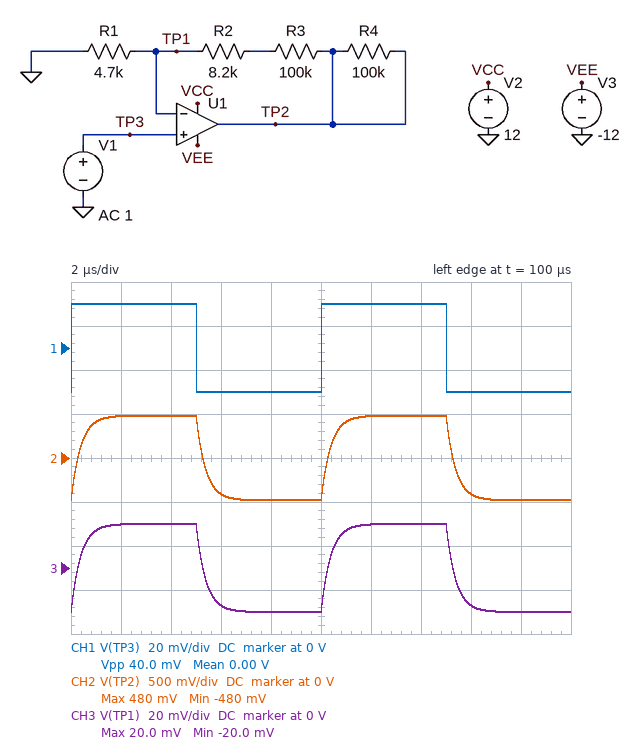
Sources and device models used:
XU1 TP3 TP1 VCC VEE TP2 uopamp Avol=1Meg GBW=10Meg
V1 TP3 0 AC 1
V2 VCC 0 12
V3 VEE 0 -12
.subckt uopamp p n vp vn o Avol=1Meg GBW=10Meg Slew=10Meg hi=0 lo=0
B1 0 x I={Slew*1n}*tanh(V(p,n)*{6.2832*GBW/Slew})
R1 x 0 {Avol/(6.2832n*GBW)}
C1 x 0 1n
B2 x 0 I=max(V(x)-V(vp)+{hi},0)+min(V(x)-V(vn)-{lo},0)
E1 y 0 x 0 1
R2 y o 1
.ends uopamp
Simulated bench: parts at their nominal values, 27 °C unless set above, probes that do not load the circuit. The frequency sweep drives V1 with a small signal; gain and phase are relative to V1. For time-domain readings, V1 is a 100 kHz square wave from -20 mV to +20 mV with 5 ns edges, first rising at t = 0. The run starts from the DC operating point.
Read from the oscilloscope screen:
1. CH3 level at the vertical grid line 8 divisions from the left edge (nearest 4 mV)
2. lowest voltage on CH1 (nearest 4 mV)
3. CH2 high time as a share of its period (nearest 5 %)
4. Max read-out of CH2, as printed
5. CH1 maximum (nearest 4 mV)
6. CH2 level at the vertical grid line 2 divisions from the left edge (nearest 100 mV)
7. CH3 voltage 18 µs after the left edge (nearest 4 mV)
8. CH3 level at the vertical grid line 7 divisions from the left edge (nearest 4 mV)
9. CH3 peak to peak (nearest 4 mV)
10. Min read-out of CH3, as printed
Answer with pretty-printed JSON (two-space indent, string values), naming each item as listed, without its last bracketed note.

{
  "CH3 level at the vertical grid line 8 divisions from the left edge": "-16 mV",
  "lowest voltage on CH1": "-20 mV",
  "CH2 high time as a share of its period": "50 %",
  "Max read-out of CH2, as printed": "480 mV",
  "CH1 maximum": "20 mV",
  "CH2 level at the vertical grid line 2 divisions from the left edge": "500 mV",
  "CH3 voltage 18 µs after the left edge": "-20 mV",
  "CH3 level at the vertical grid line 7 divisions from the left edge": "20 mV",
  "CH3 peak to peak": "40 mV",
  "Min read-out of CH3, as printed": "-20.0 mV"
}
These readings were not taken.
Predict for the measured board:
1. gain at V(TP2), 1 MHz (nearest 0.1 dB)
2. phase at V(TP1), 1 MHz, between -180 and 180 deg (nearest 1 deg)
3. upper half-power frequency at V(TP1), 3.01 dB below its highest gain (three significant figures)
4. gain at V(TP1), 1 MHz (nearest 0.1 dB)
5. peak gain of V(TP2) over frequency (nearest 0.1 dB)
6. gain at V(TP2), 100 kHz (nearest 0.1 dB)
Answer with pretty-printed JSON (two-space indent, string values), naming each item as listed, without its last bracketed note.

{
  "gain at V(TP2), 1 MHz": "19.3 dB",
  "phase at V(TP1), 1 MHz, between -180 and 180 deg": "-67 deg",
  "upper half-power frequency at V(TP1), 3.01 dB below its highest gain": "416 kHz",
  "gain at V(TP1), 1 MHz": "-8.3 dB",
  "peak gain of V(TP2) over frequency": "27.6 dB",
  "gain at V(TP2), 100 kHz": "27.4 dB"
}
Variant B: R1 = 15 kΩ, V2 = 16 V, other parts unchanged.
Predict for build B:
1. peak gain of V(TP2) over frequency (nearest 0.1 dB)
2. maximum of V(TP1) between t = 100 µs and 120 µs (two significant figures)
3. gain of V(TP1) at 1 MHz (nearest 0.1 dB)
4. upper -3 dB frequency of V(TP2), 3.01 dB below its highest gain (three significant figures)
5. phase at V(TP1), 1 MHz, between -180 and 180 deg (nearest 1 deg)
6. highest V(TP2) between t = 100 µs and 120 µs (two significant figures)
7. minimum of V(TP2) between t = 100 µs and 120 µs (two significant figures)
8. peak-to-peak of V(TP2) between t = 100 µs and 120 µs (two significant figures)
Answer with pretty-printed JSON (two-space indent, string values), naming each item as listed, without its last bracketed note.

{
  "peak gain of V(TP2) over frequency": "18.3 dB",
  "maximum of V(TP1) between t = 100 µs and 120 µs": "20 mV",
  "gain of V(TP1) at 1 MHz": "-2.2 dB",
  "upper -3 dB frequency of V(TP2), 3.01 dB below its highest gain": "1.22 MHz",
  "phase at V(TP1), 1 MHz, between -180 and 180 deg": "-39 deg",
  "highest V(TP2) between t = 100 µs and 120 µs": "160 mV",
  "minimum of V(TP2) between t = 100 µs and 120 µs": "-160 mV",
  "peak-to-peak of V(TP2) between t = 100 µs and 120 µs": "330 mV"
}
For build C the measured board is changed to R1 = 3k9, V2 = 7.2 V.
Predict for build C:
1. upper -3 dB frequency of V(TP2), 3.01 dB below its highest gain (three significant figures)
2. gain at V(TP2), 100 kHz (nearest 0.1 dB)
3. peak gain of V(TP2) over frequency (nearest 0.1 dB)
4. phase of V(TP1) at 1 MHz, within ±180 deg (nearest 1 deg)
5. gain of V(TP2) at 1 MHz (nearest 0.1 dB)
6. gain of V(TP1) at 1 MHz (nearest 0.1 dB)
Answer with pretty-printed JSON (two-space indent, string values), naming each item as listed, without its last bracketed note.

{
  "upper -3 dB frequency of V(TP2), 3.01 dB below its highest gain": "348 kHz",
  "gain at V(TP2), 100 kHz": "28.8 dB",
  "peak gain of V(TP2) over frequency": "29.2 dB",
  "phase of V(TP1) at 1 MHz, within ±180 deg": "-71 deg",
  "gain of V(TP2) at 1 MHz": "19.5 dB",
  "gain of V(TP1) at 1 MHz": "-9.7 dB"
}
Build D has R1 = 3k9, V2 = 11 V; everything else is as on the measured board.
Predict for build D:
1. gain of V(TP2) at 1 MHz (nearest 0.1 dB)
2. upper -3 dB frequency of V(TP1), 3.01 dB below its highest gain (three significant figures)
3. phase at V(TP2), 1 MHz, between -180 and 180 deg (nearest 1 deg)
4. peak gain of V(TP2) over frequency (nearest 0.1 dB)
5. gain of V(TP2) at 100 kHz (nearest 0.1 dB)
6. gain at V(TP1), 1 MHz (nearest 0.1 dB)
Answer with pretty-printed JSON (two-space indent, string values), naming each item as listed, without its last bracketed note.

{
  "gain of V(TP2) at 1 MHz": "19.5 dB",
  "upper -3 dB frequency of V(TP1), 3.01 dB below its highest gain": "348 kHz",
  "phase at V(TP2), 1 MHz, between -180 and 180 deg": "-71 deg",
  "peak gain of V(TP2) over frequency": "29.2 dB",
  "gain of V(TP2) at 100 kHz": "28.8 dB",
  "gain at V(TP1), 1 MHz": "-9.7 dB"
}
